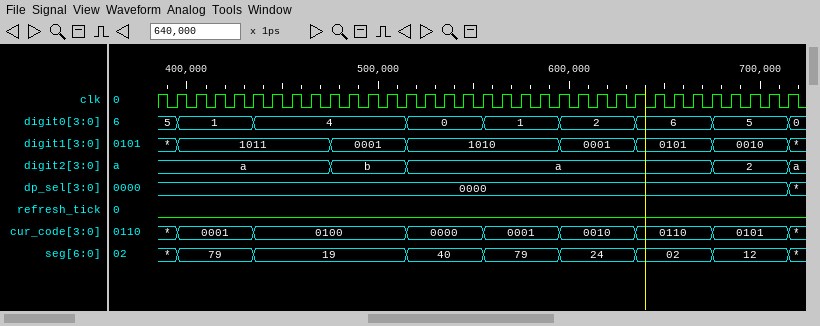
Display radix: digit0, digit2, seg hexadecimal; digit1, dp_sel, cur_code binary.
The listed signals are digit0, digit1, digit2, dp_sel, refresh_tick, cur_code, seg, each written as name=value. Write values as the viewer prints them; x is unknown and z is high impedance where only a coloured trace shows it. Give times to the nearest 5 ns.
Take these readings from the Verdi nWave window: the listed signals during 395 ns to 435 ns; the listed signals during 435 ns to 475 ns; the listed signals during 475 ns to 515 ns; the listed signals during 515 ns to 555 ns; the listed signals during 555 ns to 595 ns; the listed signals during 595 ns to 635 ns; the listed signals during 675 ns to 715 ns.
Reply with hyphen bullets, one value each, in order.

- digit0=1, digit1=1011, digit2=a, dp_sel=0000, refresh_tick=0, cur_code=0001, seg=79
- digit0=4, digit1=1011, digit2=a, dp_sel=0000, refresh_tick=0, cur_code=0100, seg=19
- digit0=4, digit1=0001, digit2=b, dp_sel=0000, refresh_tick=0, cur_code=0100, seg=19
- digit0=0, digit1=1010, digit2=a, dp_sel=0000, refresh_tick=0, cur_code=0000, seg=40
- digit0=1, digit1=1010, digit2=a, dp_sel=0000, refresh_tick=0, cur_code=0001, seg=79
- digit0=2, digit1=0001, digit2=a, dp_sel=0000, refresh_tick=0, cur_code=0010, seg=24
- digit0=5, digit1=0010, digit2=2, dp_sel=0000, refresh_tick=0, cur_code=0101, seg=12
